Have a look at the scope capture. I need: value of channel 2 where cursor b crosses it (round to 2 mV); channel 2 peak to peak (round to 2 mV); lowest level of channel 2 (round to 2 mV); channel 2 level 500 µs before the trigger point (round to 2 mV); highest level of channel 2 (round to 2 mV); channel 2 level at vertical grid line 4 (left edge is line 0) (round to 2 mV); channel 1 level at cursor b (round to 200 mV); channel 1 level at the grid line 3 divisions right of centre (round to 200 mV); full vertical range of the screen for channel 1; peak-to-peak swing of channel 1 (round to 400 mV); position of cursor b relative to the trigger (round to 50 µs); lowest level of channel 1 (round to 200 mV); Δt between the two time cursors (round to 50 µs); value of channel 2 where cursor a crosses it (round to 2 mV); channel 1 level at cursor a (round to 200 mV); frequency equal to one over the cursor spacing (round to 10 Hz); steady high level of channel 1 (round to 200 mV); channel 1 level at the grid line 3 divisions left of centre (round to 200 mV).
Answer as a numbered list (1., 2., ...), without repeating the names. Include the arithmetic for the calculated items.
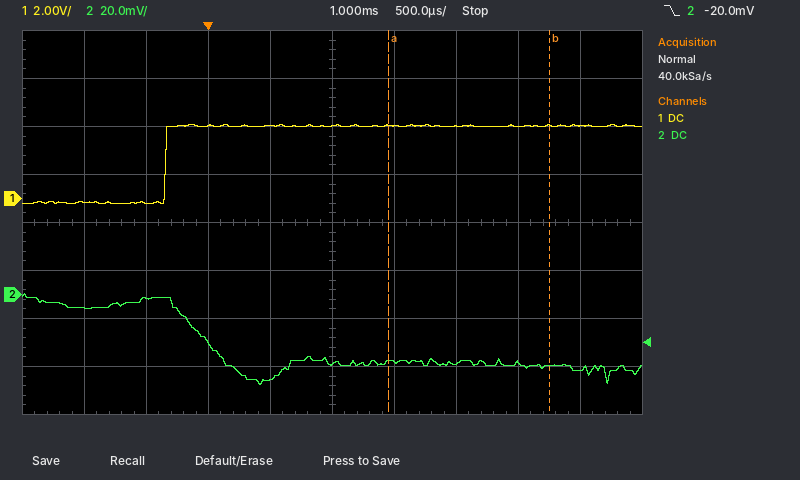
1. -30 mV
2. 0 mV − (-38 mV) = 38 mV
3. -38 mV
4. -2 mV
5. 0 mV
6. -36 mV
7. 3.0 V
8. 3.0 V
9. 16 V
10. 3.2 V
11. +2.75 ms
12. -200 mV
13. 1.30 ms
14. -28 mV
15. 3.0 V
16. 1 / 1.30 ms ≈ 770 Hz
17. 3.0 V
18. -200 mV
